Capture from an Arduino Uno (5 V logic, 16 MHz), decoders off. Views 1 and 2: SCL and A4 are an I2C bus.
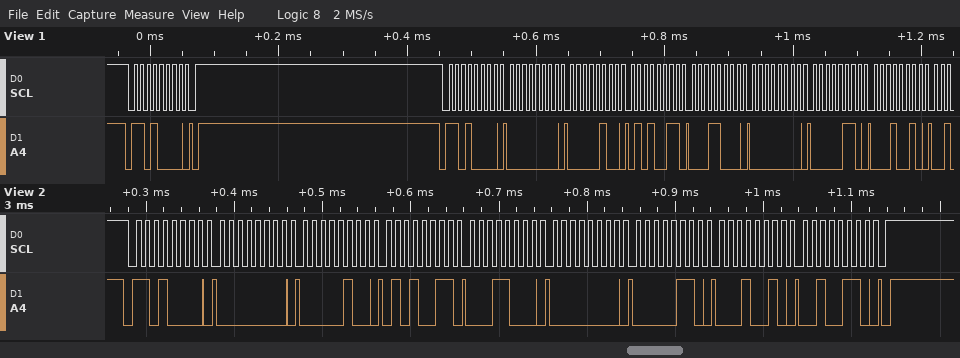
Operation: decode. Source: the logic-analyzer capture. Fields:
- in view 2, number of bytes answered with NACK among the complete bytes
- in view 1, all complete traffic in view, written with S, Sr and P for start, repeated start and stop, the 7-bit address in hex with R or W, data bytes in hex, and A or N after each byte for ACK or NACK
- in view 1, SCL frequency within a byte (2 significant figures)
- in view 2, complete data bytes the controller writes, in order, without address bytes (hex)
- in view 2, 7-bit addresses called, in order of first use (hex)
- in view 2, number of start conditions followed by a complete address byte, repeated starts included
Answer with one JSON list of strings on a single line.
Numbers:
["0", "S 68W A P S 68W A 00 A 04 A 53 A 18 A 00 A 06 A 12 A", "100 kHz", "00 04 53 18 00 06 12 26", "0x68", "1"]
